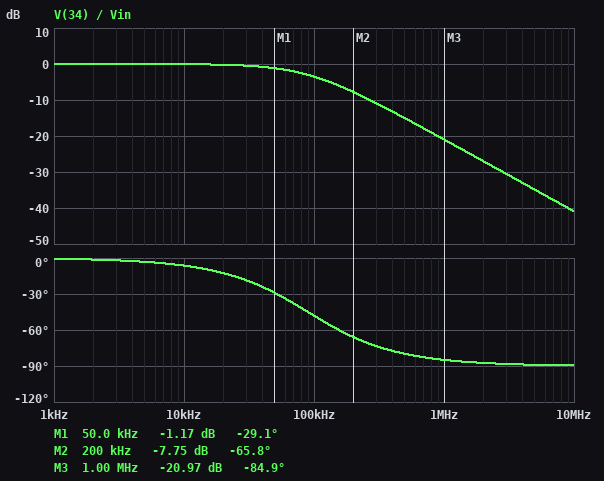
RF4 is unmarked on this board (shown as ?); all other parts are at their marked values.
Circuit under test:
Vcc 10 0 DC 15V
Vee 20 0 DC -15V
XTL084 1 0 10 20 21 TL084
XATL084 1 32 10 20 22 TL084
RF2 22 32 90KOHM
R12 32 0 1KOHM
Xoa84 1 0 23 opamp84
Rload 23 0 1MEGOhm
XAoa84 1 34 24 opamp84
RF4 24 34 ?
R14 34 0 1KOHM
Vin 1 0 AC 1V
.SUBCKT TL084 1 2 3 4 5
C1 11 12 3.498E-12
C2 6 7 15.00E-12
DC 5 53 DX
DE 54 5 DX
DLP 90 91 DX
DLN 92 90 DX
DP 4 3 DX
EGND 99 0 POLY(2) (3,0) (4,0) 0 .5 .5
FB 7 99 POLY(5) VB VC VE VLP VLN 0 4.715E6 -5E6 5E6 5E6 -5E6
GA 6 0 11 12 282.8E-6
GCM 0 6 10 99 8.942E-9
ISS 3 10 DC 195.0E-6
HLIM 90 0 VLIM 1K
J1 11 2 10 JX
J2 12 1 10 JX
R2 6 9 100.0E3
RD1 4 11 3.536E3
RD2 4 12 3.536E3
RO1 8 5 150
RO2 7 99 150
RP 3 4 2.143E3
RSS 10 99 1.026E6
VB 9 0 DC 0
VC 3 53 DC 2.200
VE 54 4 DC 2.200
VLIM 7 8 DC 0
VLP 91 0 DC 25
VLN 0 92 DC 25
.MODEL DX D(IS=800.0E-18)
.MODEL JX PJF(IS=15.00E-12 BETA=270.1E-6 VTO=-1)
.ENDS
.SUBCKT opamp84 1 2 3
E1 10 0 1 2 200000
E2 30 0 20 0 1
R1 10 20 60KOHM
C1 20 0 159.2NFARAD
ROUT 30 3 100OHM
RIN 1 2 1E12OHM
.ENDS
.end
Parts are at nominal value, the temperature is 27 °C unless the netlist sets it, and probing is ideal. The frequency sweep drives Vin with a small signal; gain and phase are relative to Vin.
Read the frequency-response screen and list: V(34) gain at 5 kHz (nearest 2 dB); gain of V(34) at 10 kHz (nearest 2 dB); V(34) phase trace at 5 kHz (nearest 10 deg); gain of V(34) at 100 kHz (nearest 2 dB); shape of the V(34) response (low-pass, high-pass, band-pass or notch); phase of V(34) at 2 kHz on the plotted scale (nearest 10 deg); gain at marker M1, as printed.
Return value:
0 dB
0 dB
0 deg
-4 dB
low-pass
0 deg
-1.17 dB
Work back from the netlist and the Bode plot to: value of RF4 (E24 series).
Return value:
36 kΩ
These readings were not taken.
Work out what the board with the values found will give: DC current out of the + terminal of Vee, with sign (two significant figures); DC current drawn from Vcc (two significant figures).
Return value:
-28 mA
28 mA
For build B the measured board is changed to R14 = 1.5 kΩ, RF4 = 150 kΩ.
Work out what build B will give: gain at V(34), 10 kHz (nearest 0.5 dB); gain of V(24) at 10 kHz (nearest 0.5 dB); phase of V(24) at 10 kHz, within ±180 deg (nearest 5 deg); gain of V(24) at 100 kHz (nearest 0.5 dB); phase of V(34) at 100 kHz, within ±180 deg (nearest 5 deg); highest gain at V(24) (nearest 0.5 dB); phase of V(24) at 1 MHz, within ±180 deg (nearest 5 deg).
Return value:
-0.5 dB
39.5 dB
-15 deg
30.0 dB
-70 deg
40.0 dB
-90 deg
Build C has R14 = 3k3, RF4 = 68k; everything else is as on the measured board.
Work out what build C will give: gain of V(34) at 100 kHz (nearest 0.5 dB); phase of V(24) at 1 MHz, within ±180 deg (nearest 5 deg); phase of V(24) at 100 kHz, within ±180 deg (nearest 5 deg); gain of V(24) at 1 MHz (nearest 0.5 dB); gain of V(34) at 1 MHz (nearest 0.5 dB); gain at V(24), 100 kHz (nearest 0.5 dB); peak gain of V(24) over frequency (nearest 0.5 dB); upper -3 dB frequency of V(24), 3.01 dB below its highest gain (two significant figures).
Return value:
-1.5 dB
-80 deg
-35 deg
10.5 dB
-16.5 dB
25.0 dB
26.5 dB
150 kHz
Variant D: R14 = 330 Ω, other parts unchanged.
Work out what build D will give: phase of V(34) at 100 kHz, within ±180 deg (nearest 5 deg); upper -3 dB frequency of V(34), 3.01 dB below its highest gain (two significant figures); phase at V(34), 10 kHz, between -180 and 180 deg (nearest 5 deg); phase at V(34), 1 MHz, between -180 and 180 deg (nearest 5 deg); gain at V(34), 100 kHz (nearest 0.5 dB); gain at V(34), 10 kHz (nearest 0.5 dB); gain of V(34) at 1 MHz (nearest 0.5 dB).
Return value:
-75 deg
30 kHz
-20 deg
-90 deg
-11.0 dB
-0.5 dB
-30.5 dB
